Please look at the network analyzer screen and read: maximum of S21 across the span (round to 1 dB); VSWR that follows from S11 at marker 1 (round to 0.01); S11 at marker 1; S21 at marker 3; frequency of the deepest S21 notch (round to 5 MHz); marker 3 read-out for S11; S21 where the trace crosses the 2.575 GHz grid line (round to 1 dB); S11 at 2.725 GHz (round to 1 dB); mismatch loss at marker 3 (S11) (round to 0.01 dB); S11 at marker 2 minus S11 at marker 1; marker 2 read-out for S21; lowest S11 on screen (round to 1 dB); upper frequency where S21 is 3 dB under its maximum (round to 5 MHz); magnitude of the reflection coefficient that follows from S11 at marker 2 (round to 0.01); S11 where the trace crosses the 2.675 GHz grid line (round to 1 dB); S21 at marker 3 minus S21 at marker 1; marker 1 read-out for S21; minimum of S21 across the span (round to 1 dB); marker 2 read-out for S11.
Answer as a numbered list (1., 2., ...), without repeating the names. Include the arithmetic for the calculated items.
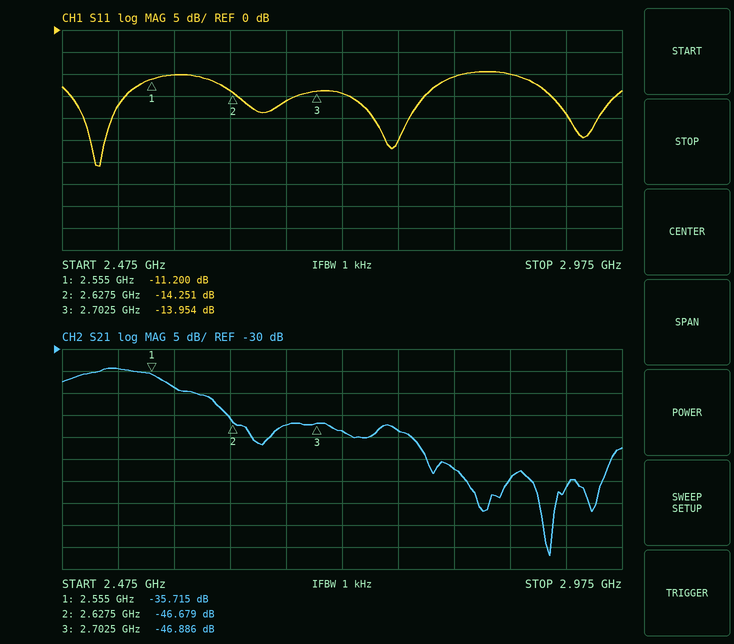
1. -34 dB
2. (1 + 0.2754)/(1 − 0.2754) ≈ 1.76
3. -11.200 dB
4. -46.886 dB
5. 2.910 GHz
6. -13.954 dB
7. -39 dB
8. -14 dB
9. −10 log10(1 − 10^(-13.954/10)) ≈ 0.18 dB
10. -14.251 − (-11.2) = -3.051 dB
11. -46.679 dB
12. -31 dB
13. 2.565 GHz
14. 10^(-14.251/20) ≈ 0.19
15. -16 dB
16. -46.886 − (-35.715) = -11.171 dB
17. -35.715 dB
18. -77 dB
19. -14.251 dB
